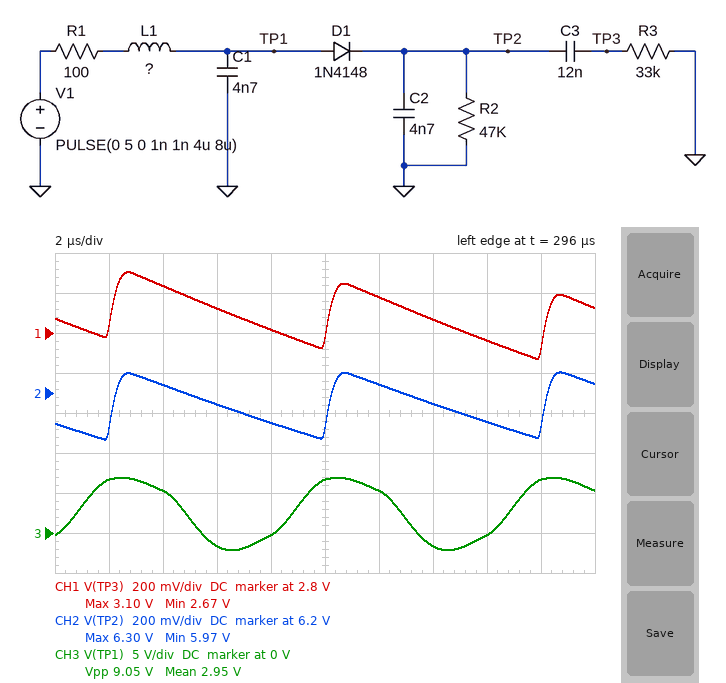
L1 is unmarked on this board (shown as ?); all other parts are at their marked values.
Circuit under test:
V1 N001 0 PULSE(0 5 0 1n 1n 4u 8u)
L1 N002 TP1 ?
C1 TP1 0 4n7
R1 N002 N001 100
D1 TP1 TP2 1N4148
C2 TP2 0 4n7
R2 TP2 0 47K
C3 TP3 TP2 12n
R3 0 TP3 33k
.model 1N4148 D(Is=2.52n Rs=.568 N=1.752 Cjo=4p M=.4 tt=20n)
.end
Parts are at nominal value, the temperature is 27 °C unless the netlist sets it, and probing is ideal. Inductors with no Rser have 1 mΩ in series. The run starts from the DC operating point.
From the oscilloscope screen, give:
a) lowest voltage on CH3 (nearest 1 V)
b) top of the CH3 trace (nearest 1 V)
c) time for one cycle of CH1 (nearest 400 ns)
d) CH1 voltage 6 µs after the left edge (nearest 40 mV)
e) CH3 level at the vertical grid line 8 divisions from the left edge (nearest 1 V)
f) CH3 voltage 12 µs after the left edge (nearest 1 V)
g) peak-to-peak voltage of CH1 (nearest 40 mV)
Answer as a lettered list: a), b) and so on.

a) -2 V
b) 7 V
c) 8.0 µs
d) 2.92 V
e) 0 V
f) 5 V
g) 440 mV
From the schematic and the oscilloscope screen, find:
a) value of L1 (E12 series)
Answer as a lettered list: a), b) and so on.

a) 150 µH
